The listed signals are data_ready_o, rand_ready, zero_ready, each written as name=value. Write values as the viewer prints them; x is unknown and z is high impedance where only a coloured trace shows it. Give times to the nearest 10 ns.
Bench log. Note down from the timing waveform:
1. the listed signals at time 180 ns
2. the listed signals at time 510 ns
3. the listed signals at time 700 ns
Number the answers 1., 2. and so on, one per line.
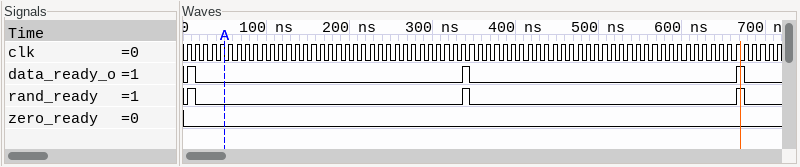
1. data_ready_o=0, rand_ready=0, zero_ready=0
2. data_ready_o=0, rand_ready=0, zero_ready=0
3. data_ready_o=0, rand_ready=0, zero_ready=0
